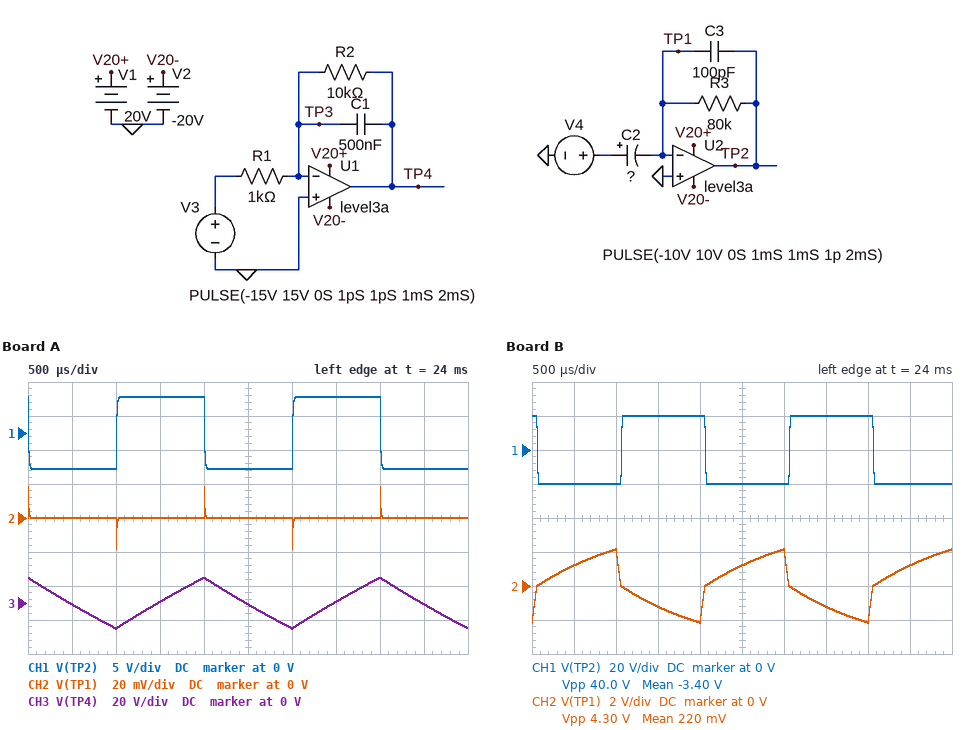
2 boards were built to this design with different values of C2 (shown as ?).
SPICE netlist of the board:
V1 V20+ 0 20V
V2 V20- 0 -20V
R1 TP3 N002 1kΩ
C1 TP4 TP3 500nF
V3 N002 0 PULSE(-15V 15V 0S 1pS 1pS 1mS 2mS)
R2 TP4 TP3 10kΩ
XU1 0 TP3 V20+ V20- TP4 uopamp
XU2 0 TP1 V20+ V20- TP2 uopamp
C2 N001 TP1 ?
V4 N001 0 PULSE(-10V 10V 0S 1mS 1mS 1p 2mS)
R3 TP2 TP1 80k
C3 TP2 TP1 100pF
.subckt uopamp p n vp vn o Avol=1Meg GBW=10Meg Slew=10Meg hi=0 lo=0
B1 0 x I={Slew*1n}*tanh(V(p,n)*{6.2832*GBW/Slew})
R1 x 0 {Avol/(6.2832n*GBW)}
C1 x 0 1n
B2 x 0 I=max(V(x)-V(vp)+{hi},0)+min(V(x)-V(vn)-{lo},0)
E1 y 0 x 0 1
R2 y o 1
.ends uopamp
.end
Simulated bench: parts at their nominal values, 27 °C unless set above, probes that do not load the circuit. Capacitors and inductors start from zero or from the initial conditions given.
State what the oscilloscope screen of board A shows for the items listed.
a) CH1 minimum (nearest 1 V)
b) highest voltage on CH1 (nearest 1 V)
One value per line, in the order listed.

-5 V
5 V
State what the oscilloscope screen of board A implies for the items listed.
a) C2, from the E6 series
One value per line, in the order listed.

3.3 nF
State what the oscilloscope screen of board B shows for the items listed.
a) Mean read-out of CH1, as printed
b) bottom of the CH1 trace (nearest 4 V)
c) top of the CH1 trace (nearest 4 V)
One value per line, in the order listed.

-3.40 V
-20 V
20 V
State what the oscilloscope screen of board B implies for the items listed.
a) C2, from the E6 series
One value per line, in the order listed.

15 nF
